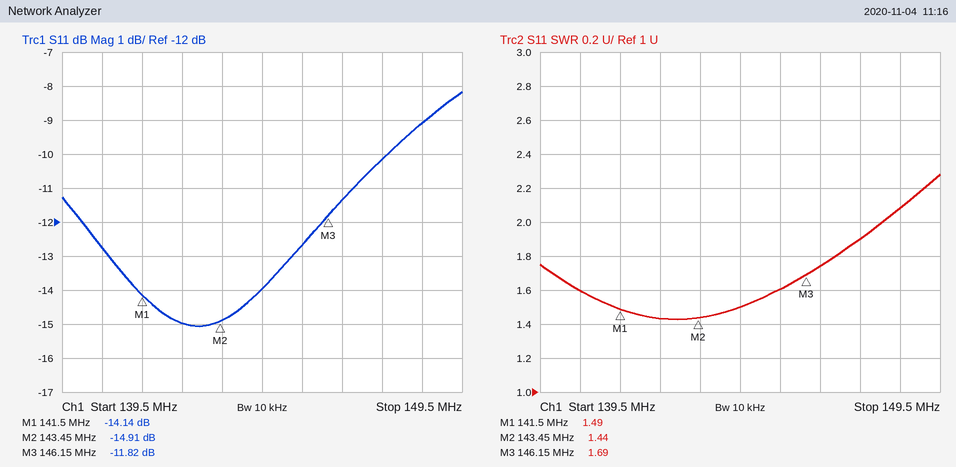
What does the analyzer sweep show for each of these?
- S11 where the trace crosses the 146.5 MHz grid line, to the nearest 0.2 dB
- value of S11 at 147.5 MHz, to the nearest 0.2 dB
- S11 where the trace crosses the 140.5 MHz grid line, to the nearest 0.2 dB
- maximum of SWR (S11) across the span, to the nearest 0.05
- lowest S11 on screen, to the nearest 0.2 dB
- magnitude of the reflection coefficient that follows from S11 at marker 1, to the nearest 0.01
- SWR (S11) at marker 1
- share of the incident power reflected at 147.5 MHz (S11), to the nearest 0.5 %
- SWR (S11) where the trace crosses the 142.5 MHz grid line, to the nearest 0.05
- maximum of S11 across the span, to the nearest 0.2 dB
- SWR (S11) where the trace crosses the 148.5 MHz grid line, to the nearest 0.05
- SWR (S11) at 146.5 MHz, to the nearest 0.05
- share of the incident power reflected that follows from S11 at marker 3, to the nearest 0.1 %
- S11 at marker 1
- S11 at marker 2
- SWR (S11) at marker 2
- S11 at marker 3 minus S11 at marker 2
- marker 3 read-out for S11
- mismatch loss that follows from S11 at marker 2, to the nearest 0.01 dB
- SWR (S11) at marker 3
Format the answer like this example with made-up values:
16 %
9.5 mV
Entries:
-11.4 dB
-10.2 dB
-12.8 dB
2.30
-15.0 dB
0.20
1.49
9.5 %
1.45
-8.2 dB
2.10
1.75
6.6 %
-14.14 dB
-14.91 dB
1.44
3.09 dB
-11.82 dB
0.14 dB
1.69
